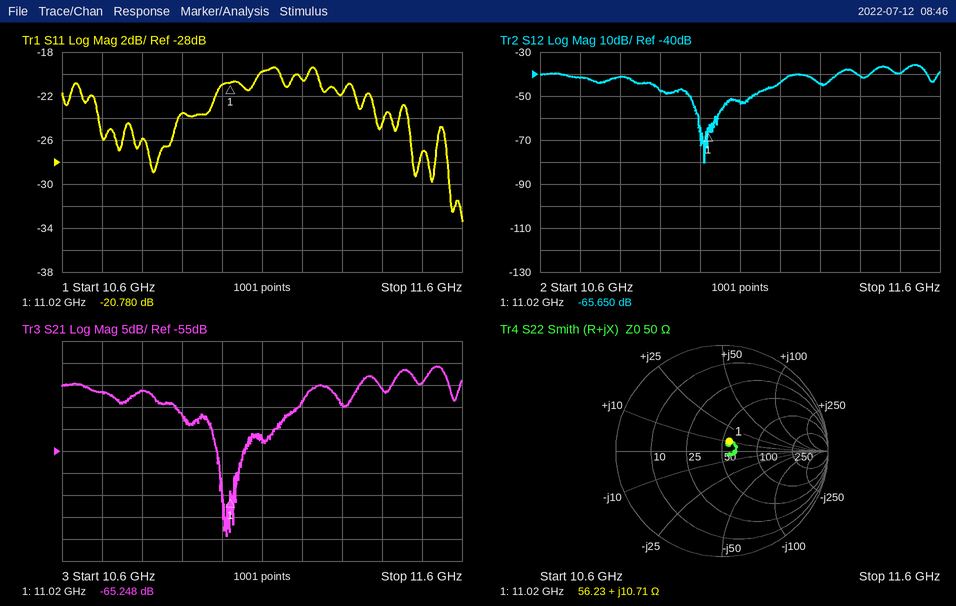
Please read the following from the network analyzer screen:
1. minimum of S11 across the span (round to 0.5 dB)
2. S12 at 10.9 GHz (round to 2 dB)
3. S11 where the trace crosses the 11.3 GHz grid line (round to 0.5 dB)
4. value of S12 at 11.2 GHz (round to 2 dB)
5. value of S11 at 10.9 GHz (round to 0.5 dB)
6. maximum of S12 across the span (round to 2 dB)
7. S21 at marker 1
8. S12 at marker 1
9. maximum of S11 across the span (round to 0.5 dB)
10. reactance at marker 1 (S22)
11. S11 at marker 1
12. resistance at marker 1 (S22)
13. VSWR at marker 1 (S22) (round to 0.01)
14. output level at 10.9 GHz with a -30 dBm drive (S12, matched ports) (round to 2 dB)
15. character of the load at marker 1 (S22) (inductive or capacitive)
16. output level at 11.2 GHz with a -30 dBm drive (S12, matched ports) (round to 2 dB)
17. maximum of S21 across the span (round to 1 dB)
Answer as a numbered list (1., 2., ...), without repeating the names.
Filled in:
1. -33.5 dB
2. -48 dB
3. -22.0 dB
4. -44 dB
5. -23.5 dB
6. -36 dB
7. -65.248 dB
8. -65.650 dB
9. -19.5 dB
10. +10.71 Ω
11. -20.780 dB
12. 56.23 Ω
13. 1.26
14. -78 dBm
15. inductive
16. -74 dBm
17. -36 dB
